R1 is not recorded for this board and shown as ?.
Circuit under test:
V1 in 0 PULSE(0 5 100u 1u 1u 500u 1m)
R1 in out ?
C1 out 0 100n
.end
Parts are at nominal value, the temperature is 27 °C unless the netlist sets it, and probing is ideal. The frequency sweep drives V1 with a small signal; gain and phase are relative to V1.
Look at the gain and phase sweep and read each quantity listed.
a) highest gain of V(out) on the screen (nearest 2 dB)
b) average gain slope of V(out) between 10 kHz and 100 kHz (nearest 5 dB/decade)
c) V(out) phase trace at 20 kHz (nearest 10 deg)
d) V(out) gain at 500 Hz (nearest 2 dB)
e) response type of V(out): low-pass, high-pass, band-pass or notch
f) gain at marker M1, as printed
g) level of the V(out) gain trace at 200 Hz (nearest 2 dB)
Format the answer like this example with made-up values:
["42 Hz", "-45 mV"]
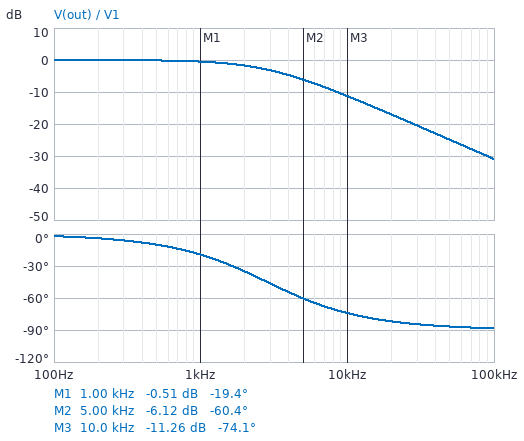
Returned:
["0 dB", "-20 dB/decade", "-80 deg", "0 dB", "low-pass", "-0.51 dB", "0 dB"]
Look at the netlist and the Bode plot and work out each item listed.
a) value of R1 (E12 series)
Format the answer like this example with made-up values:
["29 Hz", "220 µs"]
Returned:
["560 Ω"]
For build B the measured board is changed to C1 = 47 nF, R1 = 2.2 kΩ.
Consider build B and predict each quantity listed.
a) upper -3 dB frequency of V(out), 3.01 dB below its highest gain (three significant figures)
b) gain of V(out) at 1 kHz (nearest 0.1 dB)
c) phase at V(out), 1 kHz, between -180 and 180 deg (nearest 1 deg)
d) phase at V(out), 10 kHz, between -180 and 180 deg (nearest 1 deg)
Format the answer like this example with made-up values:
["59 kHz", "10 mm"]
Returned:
["1.54 kHz", "-1.5 dB", "-33 deg", "-81 deg"]
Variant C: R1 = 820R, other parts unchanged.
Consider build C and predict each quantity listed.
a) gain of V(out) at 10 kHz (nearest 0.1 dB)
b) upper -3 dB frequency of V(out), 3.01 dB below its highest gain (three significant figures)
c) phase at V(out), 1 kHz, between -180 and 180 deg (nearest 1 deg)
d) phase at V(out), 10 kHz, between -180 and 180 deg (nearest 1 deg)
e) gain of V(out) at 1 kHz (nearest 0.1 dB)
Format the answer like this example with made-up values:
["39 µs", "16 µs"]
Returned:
["-14.4 dB", "1.94 kHz", "-27 deg", "-79 deg", "-1.0 dB"]
